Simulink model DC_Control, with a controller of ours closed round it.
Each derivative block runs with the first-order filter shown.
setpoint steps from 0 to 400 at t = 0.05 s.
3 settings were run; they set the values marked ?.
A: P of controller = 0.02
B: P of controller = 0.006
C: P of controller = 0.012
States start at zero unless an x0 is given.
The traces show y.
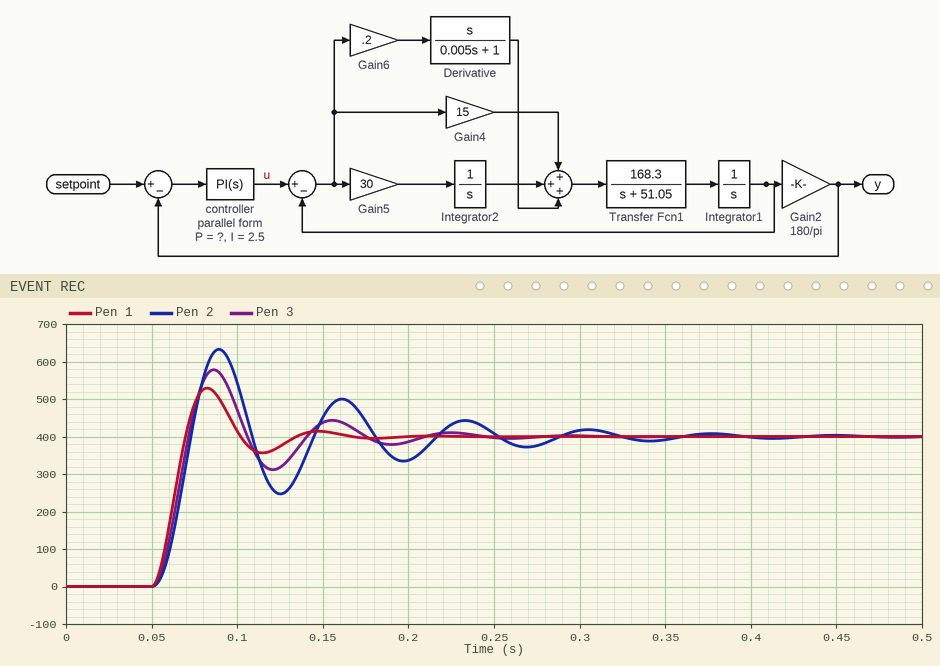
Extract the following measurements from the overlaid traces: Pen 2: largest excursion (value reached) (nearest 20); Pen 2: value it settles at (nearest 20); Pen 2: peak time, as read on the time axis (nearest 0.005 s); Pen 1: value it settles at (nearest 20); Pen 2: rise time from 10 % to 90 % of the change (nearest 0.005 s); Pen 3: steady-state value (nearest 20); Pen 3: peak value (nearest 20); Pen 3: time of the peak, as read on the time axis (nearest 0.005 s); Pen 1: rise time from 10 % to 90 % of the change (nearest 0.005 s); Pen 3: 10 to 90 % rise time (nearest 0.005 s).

640
400
0.090 s
400
0.015 s
400
580
0.085 s
0.015 s
0.015 s
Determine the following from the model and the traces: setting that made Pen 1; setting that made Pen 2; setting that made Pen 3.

A
B
C
